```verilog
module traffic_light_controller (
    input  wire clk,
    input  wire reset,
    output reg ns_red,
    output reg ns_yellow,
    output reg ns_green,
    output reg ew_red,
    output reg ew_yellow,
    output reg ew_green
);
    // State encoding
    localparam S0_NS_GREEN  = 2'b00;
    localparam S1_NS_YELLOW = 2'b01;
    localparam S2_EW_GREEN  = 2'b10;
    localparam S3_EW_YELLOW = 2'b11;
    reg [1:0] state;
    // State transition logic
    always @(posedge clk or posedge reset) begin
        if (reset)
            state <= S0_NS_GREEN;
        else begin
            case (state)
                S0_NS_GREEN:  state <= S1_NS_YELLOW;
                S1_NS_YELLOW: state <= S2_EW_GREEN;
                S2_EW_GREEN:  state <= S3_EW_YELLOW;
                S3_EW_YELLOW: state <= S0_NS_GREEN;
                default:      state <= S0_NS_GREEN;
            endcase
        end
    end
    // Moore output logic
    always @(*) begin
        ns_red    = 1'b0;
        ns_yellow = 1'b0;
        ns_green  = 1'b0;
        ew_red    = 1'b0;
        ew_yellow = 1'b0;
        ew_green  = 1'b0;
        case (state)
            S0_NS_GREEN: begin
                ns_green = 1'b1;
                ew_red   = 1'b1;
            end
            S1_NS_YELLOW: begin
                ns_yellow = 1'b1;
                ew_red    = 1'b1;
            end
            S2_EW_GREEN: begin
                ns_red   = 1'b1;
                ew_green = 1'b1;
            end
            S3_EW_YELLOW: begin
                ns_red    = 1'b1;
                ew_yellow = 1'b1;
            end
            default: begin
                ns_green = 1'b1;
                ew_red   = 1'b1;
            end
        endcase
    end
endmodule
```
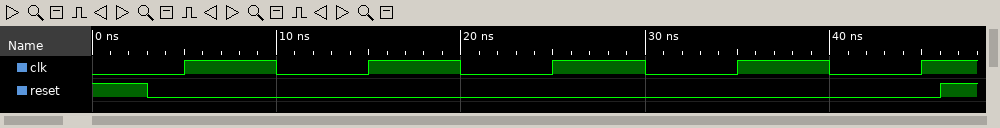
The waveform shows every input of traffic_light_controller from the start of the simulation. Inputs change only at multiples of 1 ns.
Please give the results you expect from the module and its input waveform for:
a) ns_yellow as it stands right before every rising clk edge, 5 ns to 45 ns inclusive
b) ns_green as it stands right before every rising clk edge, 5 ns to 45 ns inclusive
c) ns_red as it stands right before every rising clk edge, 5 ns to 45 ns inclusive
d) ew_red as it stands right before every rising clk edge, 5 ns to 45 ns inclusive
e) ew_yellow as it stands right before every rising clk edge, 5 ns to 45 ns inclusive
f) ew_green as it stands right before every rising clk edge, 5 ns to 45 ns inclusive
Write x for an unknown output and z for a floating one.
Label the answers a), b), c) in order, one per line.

a) 0 1 0 0 0
b) 1 0 0 0 1
c) 0 0 1 1 0
d) 1 1 0 0 1
e) 0 0 0 1 0
f) 0 0 1 0 0
